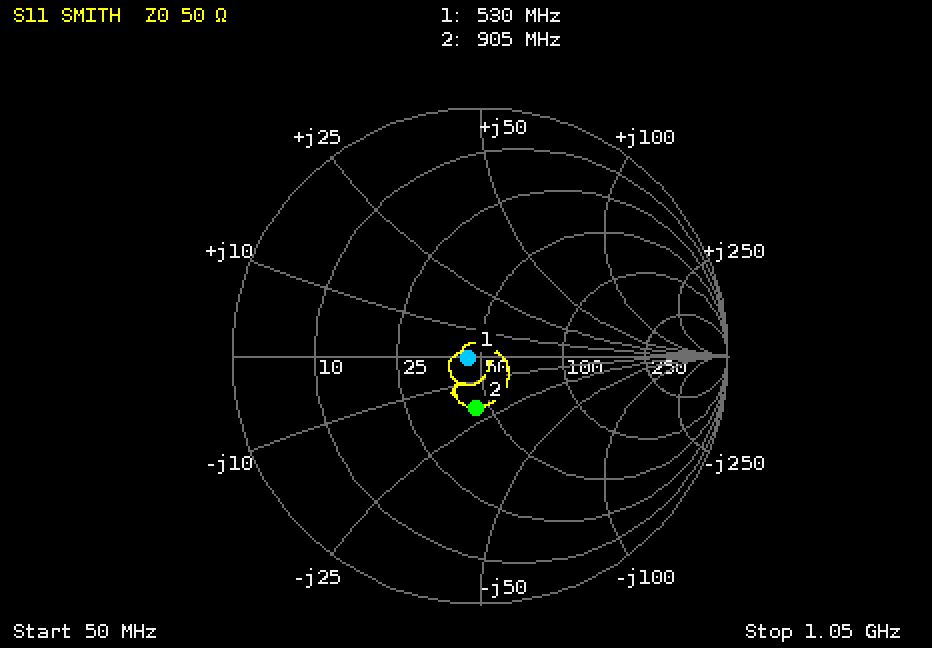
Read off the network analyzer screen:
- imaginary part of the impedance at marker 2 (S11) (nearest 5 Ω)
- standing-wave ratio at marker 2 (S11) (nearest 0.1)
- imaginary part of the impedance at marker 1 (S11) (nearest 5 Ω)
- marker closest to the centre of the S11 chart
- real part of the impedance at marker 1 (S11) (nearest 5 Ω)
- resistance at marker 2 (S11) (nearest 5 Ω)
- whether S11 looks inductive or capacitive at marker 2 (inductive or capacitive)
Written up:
-20 Ω
1.5
0 Ω
marker 1
45 Ω
45 Ω
capacitive
